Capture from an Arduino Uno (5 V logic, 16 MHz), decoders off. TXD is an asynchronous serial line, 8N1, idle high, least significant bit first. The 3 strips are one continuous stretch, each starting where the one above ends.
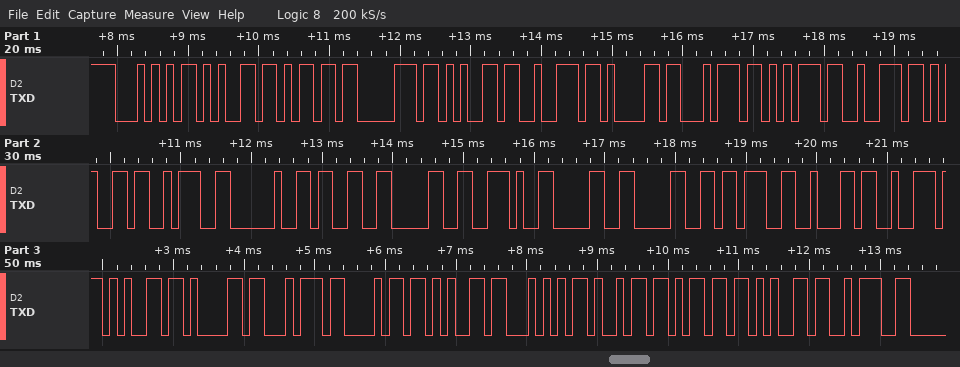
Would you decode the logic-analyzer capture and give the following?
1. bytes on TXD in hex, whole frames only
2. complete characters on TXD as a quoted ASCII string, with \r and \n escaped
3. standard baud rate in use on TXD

0x54 0x65 0x6D 0x70 0x65 0x72 0x61 0x74 0x75 0x72 0x65 0x3A 0x20 0x33 0x30 0x2E 0x30 0x30 0x3B 0x62 0x72 0x65 0x61 0x74 0x68 0x65 0x54 0x69 0x6D 0x65 0x3A
"Temperature: 30.00;breatheTime:"
9600 baud
